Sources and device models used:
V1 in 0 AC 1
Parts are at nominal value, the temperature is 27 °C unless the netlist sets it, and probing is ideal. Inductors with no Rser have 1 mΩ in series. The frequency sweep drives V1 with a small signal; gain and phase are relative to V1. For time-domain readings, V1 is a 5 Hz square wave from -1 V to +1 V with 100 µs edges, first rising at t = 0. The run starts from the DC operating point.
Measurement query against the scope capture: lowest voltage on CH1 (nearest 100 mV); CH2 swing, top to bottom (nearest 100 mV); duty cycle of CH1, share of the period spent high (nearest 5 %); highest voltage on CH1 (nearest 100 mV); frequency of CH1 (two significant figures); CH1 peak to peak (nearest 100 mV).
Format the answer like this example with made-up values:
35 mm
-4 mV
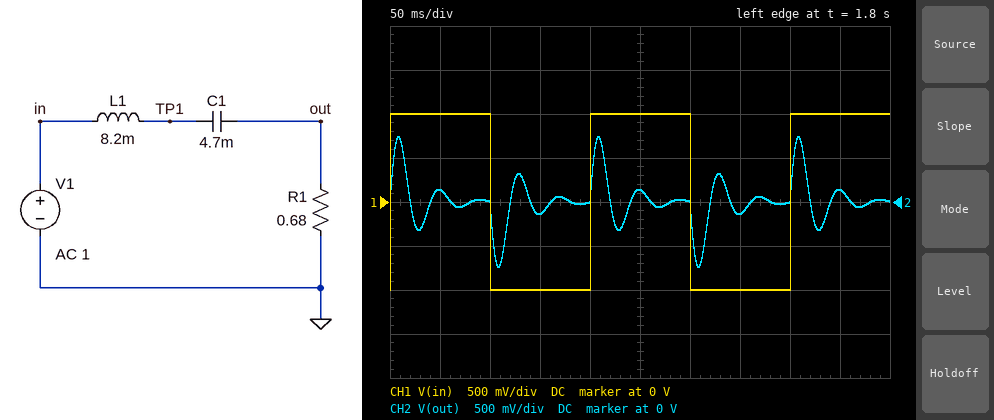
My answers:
-1.0 V
1.5 V
50 %
1.0 V
5.0 Hz
2.0 V
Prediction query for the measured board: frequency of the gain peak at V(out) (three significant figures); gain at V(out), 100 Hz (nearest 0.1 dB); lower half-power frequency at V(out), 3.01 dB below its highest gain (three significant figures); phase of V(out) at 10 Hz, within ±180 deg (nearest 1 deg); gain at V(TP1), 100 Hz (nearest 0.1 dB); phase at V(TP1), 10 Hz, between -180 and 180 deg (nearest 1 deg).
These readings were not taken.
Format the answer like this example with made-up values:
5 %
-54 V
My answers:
25.6 Hz
-17.1 dB
19.9 Hz
77 deg
-16.1 dB
-2 deg
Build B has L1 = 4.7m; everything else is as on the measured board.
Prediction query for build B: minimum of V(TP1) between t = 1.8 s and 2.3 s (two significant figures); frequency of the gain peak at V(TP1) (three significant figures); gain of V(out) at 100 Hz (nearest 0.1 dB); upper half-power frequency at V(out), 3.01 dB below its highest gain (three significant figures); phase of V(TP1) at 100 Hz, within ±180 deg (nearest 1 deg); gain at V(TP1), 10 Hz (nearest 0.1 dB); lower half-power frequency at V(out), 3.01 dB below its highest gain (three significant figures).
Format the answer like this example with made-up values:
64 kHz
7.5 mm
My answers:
-1.8 V
31.0 Hz
-12.0 dB
47.3 Hz
-102 deg
0.8 dB
24.2 Hz
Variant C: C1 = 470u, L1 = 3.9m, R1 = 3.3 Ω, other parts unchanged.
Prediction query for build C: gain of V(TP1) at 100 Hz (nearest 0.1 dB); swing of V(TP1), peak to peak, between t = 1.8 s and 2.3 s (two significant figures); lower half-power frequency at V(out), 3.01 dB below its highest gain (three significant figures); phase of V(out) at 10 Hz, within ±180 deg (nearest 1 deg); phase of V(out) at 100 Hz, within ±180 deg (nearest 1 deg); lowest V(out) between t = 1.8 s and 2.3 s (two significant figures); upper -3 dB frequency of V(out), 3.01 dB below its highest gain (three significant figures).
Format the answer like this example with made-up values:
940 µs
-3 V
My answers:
2.8 dB
3.1 V
68.1 Hz
84 deg
16 deg
-1.2 V
203 Hz
